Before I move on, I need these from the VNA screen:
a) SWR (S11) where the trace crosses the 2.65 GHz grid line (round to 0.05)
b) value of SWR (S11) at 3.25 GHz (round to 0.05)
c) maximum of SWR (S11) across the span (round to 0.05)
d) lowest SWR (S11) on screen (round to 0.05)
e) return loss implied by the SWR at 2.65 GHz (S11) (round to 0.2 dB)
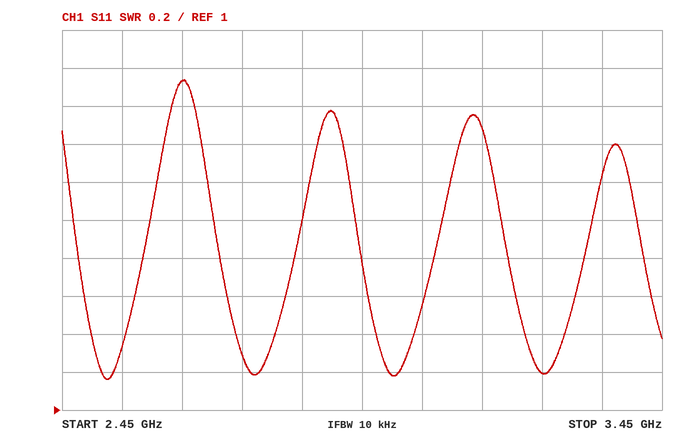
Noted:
2.75
1.20
2.75
1.15
6.6 dB
